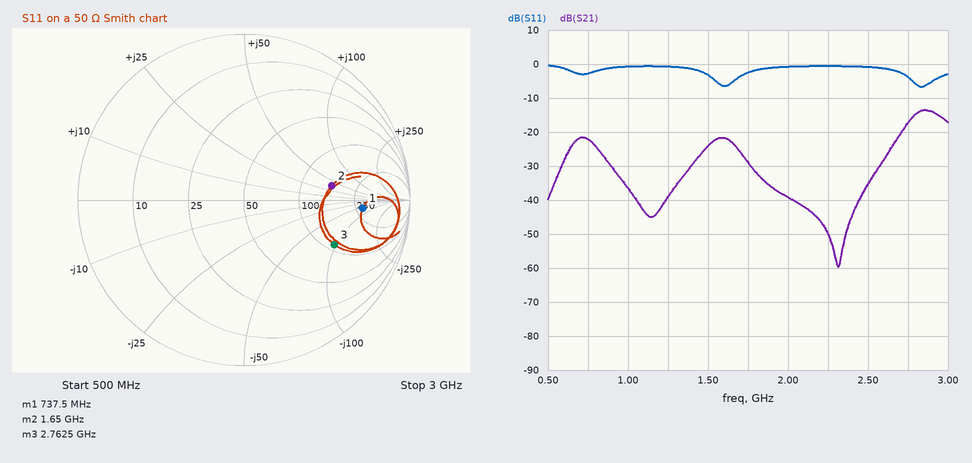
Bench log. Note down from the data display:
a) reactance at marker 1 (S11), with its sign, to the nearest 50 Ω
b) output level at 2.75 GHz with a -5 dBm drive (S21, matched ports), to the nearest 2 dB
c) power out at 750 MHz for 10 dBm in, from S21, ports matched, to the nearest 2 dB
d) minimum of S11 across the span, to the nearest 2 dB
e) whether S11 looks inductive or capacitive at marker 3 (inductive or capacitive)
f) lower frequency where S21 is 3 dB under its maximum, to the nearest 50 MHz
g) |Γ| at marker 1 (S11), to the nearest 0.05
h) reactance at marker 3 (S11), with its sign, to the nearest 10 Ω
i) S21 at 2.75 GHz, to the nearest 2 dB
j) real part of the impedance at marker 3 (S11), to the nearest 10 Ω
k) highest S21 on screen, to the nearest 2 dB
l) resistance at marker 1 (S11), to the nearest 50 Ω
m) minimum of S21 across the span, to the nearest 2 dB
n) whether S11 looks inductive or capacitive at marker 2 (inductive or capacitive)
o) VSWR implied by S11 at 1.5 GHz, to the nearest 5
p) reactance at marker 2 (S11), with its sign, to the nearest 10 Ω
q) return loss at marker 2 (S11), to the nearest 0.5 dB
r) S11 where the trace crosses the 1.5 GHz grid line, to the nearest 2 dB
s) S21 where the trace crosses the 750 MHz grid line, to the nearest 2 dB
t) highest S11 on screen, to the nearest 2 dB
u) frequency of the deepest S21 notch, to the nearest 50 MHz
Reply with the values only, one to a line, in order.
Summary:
-50 Ω
-22 dBm
-12 dBm
-6 dB
capacitive
2.75 GHz
0.70
-100 Ω
-18 dB
110 Ω
-14 dB
300 Ω
-60 dB
inductive
5
+40 Ω
5.5 dB
-4 dB
-22 dB
0 dB
2.30 GHz
